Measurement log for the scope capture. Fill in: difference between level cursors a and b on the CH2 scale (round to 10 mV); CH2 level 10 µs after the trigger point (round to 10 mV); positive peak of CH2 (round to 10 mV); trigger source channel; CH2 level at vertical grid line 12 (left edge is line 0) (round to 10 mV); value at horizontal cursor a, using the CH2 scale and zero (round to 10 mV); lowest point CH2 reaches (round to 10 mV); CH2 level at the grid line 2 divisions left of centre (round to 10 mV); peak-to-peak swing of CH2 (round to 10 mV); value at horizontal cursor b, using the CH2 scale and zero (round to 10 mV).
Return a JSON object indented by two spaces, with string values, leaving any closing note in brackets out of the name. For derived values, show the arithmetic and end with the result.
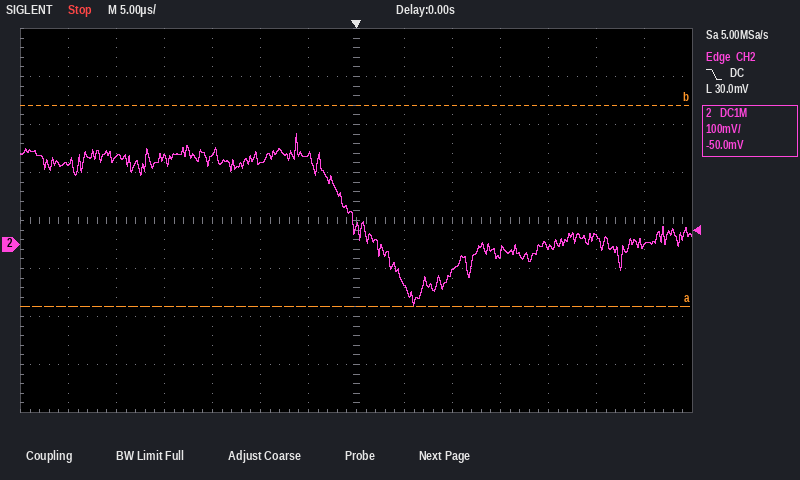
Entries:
{
  "difference between level cursors a and b on the CH2 scale": "420 mV",
  "CH2 level 10 µs after the trigger point": "-60 mV",
  "positive peak of CH2": "230 mV",
  "trigger source channel": "CH2",
  "CH2 level at vertical grid line 12 (left edge is line 0)": "20 mV",
  "value at horizontal cursor a, using the CH2 scale and zero": "-130 mV",
  "lowest point CH2 reaches": "-130 mV",
  "CH2 level at the grid line 2 divisions left of centre": "170 mV",
  "peak-to-peak swing of CH2": "230 mV − (-130 mV) = 360 mV",
  "value at horizontal cursor b, using the CH2 scale and zero": "290 mV"
}
